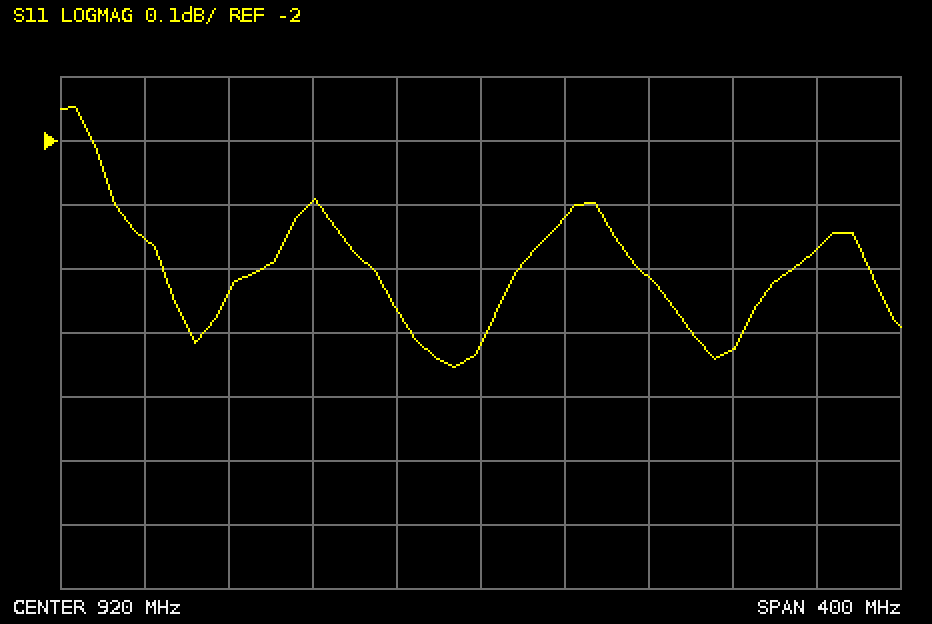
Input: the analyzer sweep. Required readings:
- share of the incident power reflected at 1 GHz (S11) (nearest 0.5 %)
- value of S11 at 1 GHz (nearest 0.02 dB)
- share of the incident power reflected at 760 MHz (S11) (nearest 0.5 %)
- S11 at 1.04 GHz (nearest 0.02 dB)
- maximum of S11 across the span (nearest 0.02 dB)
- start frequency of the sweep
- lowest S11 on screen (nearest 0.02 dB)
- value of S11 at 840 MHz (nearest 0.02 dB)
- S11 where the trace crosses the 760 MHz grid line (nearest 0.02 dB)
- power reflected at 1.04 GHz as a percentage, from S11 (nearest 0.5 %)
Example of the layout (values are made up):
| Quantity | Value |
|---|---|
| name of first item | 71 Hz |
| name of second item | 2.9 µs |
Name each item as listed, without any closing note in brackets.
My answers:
| Quantity | Value |
|---|---|
| share of the incident power reflected at 1 GHz (S11) | 60.0 % |
| value of S11 at 1 GHz | -2.22 dB |
| share of the incident power reflected at 760 MHz (S11) | 61.0 % |
| S11 at 1.04 GHz | -2.32 dB |
| maximum of S11 across the span | -1.94 dB |
| start frequency of the sweep | 720 MHz |
| lowest S11 on screen | -2.36 dB |
| value of S11 at 840 MHz | -2.10 dB |
| S11 where the trace crosses the 760 MHz grid line | -2.16 dB |
| power reflected at 1.04 GHz as a percentage, from S11 | 58.5 % |
